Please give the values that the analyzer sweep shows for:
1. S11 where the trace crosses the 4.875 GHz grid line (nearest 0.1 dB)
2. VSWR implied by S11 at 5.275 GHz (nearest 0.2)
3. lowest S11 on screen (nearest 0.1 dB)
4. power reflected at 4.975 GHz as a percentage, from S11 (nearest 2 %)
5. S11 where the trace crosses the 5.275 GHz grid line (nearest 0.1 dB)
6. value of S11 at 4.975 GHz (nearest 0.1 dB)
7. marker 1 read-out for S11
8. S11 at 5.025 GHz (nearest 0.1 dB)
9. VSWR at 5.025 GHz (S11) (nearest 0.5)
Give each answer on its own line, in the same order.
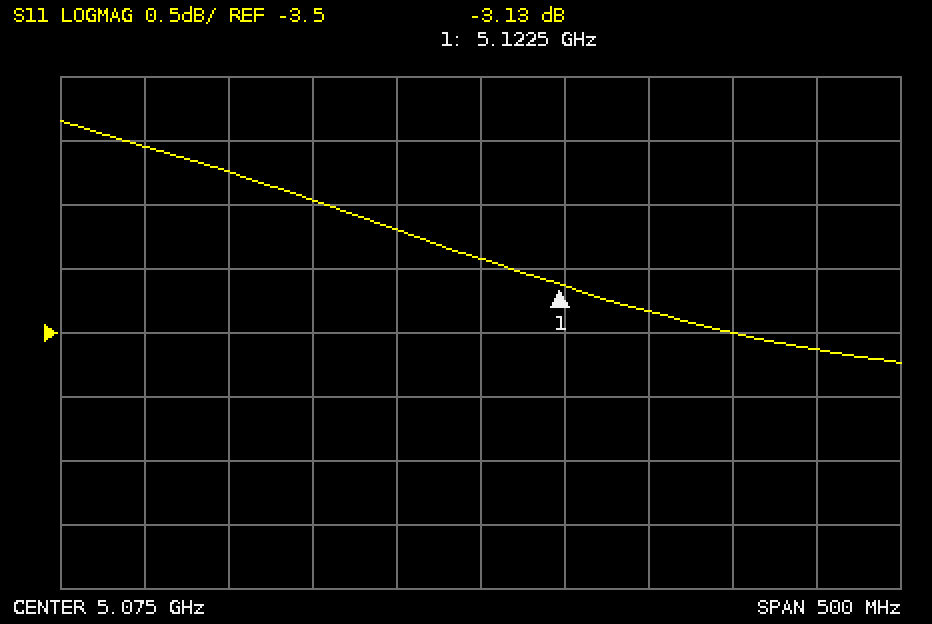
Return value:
-2.0 dB
4.8
-3.7 dB
56 %
-3.6 dB
-2.5 dB
-3.13 dB
-2.7 dB
6.5
